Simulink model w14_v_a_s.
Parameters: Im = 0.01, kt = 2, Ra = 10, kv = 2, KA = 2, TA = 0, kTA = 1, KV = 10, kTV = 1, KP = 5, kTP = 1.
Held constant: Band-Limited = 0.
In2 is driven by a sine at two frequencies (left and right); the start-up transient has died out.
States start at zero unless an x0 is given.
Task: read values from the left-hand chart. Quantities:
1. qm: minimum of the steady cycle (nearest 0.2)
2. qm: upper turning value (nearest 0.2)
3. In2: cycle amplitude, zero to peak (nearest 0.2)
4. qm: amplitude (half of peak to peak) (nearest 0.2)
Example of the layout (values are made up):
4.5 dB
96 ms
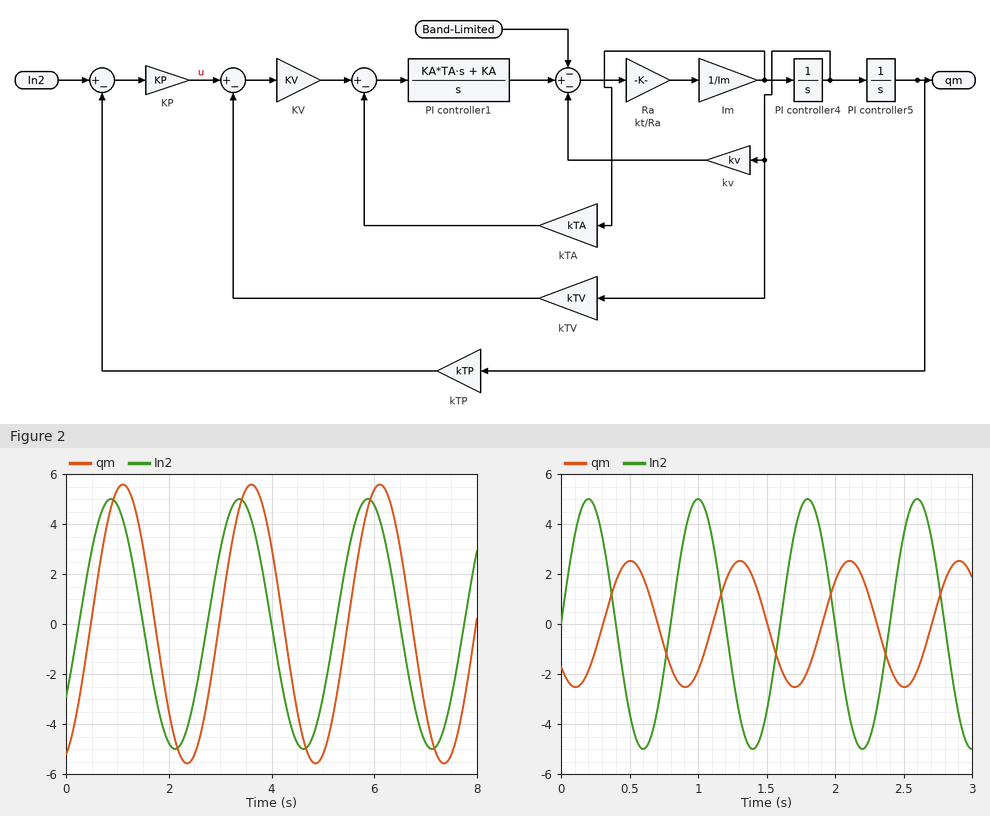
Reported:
-5.6
5.6
5.0
5.6
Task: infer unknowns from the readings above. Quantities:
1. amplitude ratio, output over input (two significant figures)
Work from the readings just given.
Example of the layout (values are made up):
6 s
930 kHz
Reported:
1.1
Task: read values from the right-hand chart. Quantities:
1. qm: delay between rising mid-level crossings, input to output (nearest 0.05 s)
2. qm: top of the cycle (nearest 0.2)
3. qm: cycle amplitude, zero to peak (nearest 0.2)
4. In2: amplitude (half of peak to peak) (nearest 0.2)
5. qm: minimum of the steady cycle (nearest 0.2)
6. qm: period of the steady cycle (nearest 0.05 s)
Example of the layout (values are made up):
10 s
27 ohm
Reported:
0.30 s
2.6
2.6
5.0
-2.6
0.80 s
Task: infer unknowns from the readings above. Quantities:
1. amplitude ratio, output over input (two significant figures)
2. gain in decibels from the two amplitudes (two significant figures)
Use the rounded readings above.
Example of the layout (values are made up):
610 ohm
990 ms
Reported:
0.52
-5.7 dB
